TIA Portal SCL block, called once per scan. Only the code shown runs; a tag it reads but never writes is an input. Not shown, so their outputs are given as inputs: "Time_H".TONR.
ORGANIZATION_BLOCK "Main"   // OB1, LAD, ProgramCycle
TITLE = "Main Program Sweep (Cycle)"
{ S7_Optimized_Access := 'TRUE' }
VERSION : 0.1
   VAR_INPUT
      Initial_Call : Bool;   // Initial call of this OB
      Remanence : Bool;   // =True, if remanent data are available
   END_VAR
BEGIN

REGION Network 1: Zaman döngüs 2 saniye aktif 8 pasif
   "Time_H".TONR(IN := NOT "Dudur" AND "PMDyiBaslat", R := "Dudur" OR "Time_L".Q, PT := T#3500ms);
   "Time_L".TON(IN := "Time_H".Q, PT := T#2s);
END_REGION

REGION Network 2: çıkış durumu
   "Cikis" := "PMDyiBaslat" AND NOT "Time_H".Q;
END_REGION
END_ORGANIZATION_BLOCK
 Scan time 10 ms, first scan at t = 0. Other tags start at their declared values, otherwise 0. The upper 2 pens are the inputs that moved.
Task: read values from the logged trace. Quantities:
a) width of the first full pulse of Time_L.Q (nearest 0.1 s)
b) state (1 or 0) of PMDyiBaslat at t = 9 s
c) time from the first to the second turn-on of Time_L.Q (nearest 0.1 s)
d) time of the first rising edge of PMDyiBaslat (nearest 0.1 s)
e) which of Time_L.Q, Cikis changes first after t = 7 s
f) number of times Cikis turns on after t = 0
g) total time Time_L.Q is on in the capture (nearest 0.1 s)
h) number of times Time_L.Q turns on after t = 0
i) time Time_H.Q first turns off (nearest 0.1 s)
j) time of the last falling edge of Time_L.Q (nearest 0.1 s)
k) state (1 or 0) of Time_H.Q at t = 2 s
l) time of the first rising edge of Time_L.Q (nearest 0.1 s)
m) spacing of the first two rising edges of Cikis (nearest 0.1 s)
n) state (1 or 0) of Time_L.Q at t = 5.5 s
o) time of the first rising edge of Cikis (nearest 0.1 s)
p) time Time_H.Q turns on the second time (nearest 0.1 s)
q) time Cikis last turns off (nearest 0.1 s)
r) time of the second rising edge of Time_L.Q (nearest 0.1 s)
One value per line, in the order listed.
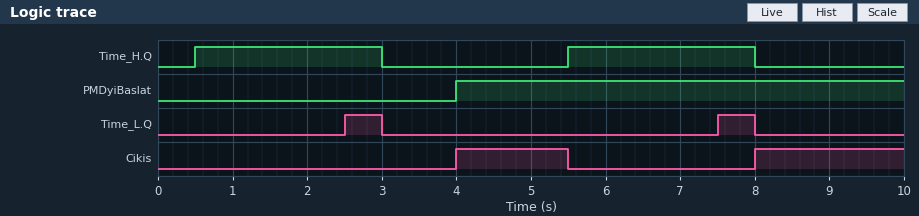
0.5 s
1
5.0 s
4.0 s
Time_L.Q
2
1.0 s
2
3.0 s
8.0 s
1
2.5 s
4.0 s
0
4.0 s
5.5 s
5.5 s
7.5 s
